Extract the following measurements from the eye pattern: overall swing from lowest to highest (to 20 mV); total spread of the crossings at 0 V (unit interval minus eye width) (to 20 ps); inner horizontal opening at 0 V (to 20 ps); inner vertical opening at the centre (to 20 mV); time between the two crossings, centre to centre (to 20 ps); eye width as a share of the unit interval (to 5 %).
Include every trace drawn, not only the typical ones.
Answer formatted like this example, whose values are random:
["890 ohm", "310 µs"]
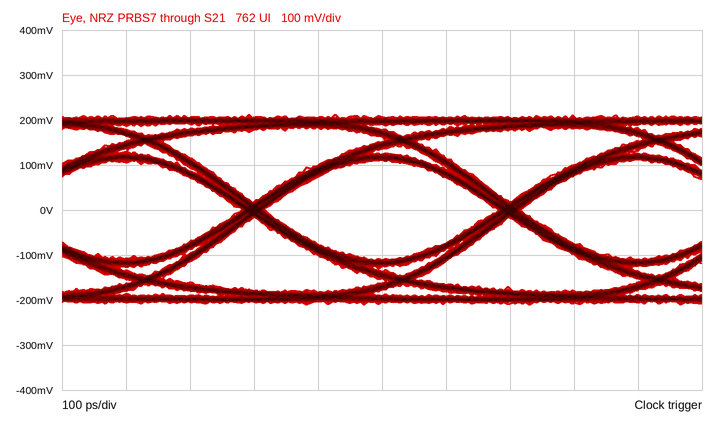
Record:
["420 mV", "40 ps", "360 ps", "220 mV", "400 ps", "90 %"]
